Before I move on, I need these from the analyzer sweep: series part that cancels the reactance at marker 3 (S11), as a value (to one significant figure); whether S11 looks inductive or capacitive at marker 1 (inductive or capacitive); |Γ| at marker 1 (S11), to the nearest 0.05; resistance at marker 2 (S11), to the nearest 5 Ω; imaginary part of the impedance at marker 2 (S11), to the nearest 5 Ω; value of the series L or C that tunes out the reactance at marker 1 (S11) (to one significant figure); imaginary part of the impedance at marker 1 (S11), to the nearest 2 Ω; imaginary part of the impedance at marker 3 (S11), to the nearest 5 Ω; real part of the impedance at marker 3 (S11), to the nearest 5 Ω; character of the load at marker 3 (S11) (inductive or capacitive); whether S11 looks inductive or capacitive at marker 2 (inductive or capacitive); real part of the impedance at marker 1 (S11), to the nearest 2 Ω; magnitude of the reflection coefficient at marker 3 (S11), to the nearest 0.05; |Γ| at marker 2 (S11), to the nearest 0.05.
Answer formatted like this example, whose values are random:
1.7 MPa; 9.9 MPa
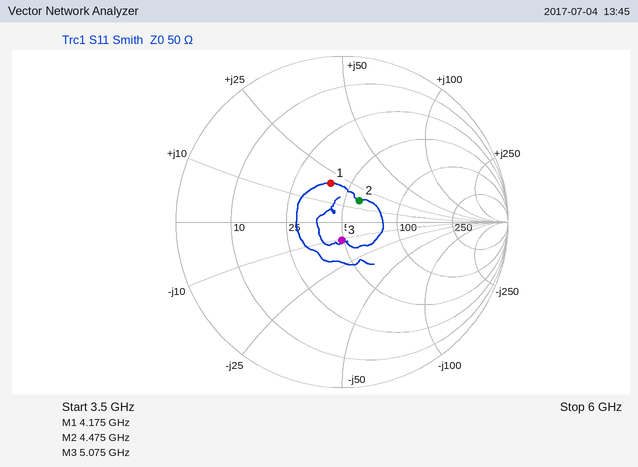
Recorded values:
300 pH; inductive; 0.25; 60 Ω; +15 Ω; 2 pF; +20 Ω; -10 Ω; 50 Ω; capacitive; inductive; 40 Ω; 0.10; 0.15
